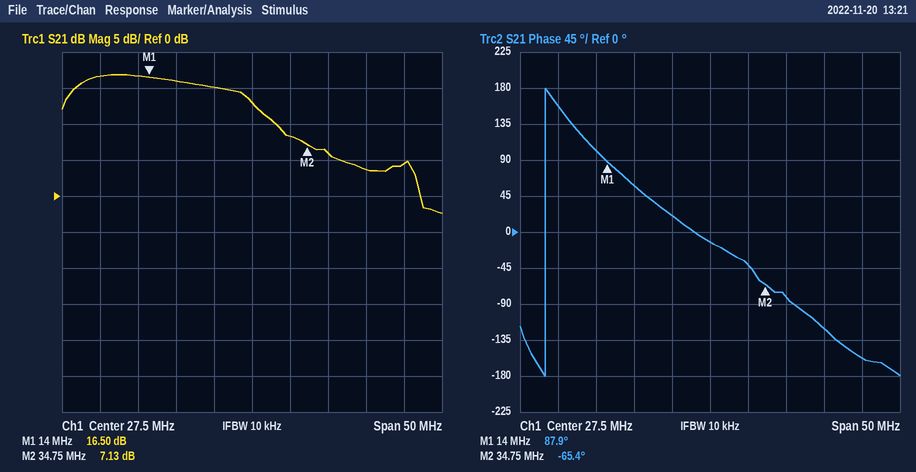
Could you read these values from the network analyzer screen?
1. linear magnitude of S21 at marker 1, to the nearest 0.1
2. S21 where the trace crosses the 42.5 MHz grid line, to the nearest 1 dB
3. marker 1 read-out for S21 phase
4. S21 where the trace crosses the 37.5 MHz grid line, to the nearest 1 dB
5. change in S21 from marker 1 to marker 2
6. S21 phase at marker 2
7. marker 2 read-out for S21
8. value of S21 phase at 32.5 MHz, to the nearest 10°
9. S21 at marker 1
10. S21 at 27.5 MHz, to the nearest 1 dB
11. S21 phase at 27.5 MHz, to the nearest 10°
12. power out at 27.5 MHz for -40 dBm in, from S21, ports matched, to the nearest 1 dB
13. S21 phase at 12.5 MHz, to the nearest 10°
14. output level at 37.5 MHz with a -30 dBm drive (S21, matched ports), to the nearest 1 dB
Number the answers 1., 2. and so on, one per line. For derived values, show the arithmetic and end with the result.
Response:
1. 10^(16.5/20) ≈ 6.7
2. 4 dB
3. 87.9°
4. 6 dB
5. 7.13 − (16.5) = -9.37 dB
6. -65.4°
7. 7.13 dB
8. -40°
9. 16.50 dB
10. 13 dB
11. -10°
12. -40 dBm + (13 dB) = -27 dBm
13. 100°
14. -30 dBm + (6 dB) = -24 dBm
